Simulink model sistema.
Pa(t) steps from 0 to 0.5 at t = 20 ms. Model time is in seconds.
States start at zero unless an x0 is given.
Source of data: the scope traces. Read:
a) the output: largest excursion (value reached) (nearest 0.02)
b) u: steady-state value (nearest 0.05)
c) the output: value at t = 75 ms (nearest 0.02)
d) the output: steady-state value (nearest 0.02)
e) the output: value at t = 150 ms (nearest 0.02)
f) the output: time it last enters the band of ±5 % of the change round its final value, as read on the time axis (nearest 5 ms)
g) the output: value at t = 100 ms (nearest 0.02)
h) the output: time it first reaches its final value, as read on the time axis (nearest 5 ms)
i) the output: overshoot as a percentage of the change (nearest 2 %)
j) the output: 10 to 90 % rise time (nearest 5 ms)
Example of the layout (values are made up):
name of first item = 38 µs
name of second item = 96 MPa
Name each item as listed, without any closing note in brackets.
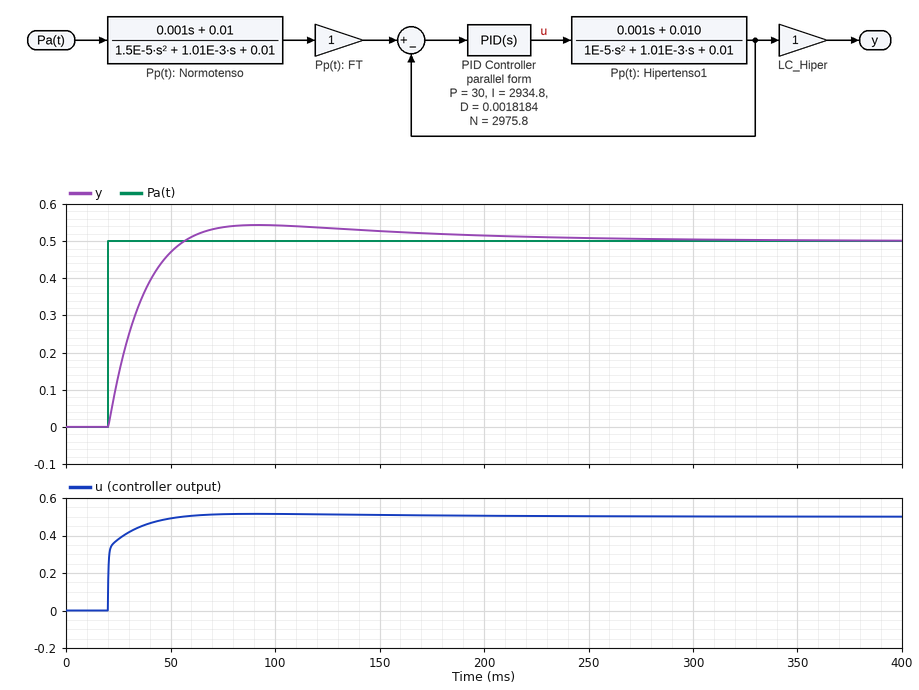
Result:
the output: largest excursion (value reached) = 0.54
u: steady-state value = 0.50
the output: value at t = 75 ms = 0.54
the output: steady-state value = 0.50
the output: value at t = 150 ms = 0.52
the output: time it last enters the band of ±5 % of the change round its final value, as read on the time axis = 155 ms
the output: value at t = 100 ms = 0.54
the output: time it first reaches its final value, as read on the time axis = 55 ms
the output: overshoot as a percentage of the change = 8 %
the output: 10 to 90 % rise time = 25 ms
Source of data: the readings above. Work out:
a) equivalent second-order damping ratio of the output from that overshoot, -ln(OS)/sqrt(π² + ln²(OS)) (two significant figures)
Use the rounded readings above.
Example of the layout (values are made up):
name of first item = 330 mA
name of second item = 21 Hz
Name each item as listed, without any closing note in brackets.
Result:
equivalent second-order damping ratio of the output from that overshoot, -ln(OS)/sqrt(π² + ln²(OS)) = 0.63
